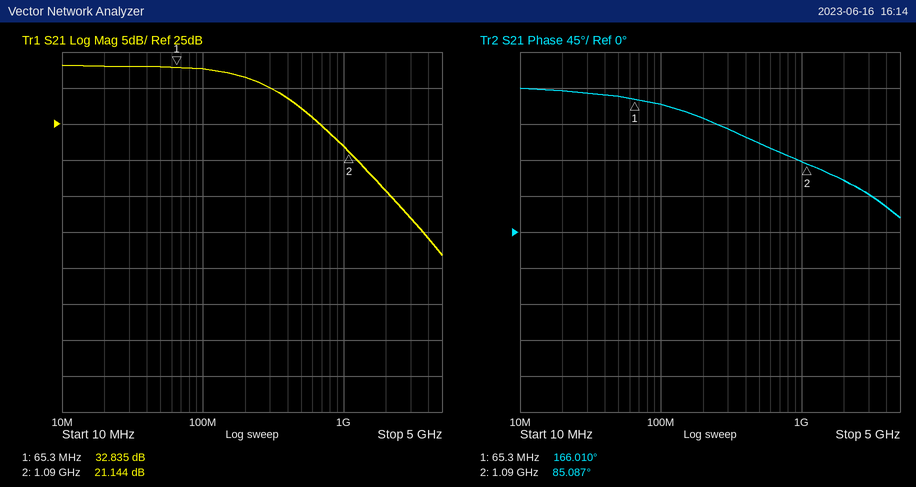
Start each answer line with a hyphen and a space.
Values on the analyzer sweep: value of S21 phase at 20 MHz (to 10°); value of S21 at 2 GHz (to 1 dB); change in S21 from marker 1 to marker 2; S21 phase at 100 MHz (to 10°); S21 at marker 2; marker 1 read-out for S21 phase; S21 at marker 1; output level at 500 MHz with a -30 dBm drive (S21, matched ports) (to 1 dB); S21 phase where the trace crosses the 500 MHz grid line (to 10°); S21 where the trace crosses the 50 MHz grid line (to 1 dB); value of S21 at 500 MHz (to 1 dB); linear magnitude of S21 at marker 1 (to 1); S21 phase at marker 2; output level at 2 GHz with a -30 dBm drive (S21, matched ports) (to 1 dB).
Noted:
- 180°
- 16 dB
- -11.691 dB
- 160°
- 21.144 dB
- 166.010°
- 32.835 dB
- -3 dBm
- 110°
- 33 dB
- 27 dB
- 44
- 85.087°
- -14 dBm
